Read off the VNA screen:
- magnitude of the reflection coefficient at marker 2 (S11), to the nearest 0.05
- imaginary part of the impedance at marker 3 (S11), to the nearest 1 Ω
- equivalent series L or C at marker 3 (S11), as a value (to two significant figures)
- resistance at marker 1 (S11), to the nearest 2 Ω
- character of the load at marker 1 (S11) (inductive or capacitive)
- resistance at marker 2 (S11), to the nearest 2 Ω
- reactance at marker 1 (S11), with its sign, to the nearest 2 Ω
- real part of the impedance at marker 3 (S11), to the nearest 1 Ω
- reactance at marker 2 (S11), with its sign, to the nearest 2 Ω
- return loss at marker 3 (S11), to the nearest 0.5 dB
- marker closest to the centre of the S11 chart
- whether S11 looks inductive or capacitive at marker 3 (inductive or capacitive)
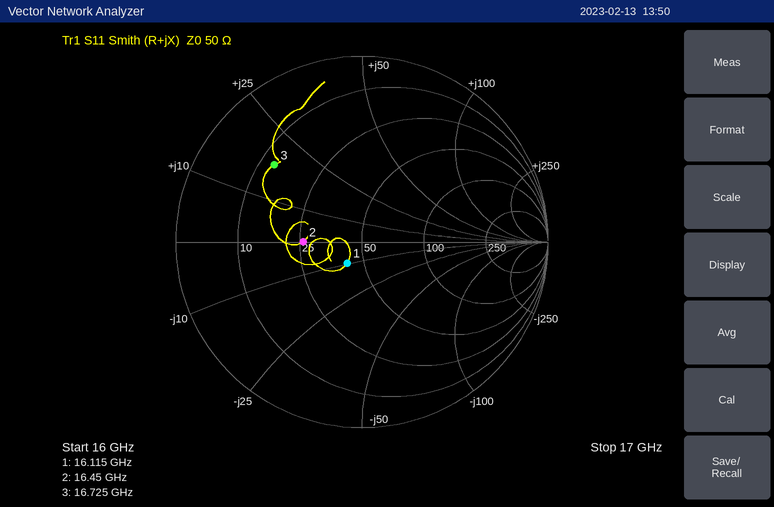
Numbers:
0.30
+18 Ω
170 pH
42 Ω
capacitive
26 Ω
-10 Ω
13 Ω
0 Ω
4.0 dB
marker 1
inductive
